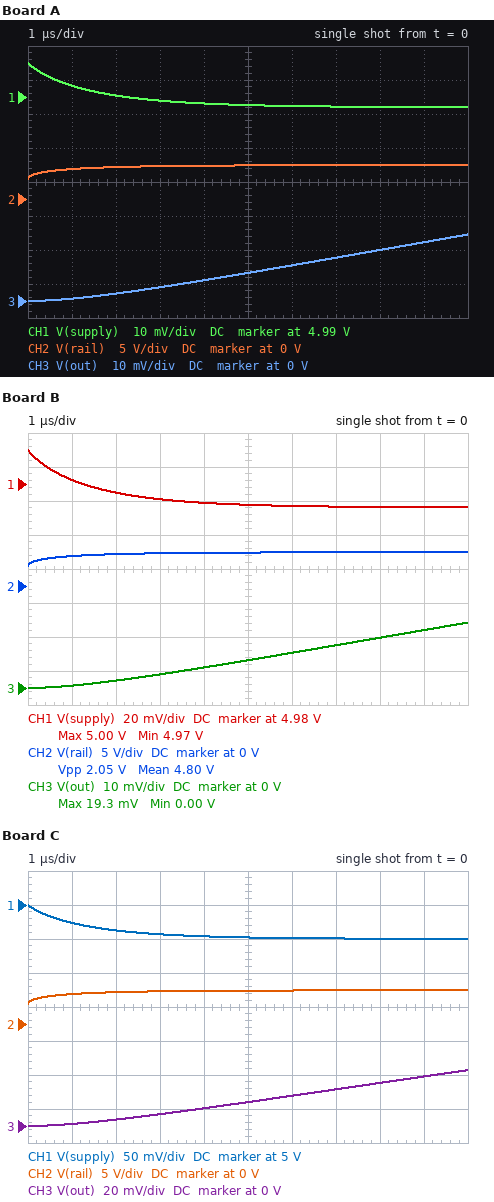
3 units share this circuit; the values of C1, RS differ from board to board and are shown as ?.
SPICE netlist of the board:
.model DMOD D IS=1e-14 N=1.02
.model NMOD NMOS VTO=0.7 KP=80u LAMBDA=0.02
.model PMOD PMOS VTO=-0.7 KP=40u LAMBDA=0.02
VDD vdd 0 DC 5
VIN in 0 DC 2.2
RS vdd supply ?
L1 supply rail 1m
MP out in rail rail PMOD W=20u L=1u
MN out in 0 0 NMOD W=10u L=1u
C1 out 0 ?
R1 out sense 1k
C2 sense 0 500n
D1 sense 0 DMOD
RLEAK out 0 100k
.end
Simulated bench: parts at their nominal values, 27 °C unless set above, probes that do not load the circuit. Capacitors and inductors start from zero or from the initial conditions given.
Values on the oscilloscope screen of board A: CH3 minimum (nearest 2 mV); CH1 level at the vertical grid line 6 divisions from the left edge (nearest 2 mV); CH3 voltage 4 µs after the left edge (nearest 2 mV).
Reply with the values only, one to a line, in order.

0 V
4.988 V
6 mV
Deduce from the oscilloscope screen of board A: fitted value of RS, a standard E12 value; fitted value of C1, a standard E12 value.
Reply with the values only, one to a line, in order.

6.8 Ω
820 nF
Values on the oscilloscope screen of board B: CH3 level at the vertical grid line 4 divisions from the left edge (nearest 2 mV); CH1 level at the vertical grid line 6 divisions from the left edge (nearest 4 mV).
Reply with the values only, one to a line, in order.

6 mV
4.968 V
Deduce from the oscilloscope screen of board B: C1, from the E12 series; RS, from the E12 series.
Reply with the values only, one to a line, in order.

820 nF
18 Ω
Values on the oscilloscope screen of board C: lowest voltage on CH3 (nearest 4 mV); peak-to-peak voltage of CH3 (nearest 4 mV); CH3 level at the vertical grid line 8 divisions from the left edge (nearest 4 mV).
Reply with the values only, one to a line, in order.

0 V
32 mV
24 mV
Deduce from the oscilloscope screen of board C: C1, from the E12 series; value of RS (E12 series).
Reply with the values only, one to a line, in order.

470 nF
27 Ω
